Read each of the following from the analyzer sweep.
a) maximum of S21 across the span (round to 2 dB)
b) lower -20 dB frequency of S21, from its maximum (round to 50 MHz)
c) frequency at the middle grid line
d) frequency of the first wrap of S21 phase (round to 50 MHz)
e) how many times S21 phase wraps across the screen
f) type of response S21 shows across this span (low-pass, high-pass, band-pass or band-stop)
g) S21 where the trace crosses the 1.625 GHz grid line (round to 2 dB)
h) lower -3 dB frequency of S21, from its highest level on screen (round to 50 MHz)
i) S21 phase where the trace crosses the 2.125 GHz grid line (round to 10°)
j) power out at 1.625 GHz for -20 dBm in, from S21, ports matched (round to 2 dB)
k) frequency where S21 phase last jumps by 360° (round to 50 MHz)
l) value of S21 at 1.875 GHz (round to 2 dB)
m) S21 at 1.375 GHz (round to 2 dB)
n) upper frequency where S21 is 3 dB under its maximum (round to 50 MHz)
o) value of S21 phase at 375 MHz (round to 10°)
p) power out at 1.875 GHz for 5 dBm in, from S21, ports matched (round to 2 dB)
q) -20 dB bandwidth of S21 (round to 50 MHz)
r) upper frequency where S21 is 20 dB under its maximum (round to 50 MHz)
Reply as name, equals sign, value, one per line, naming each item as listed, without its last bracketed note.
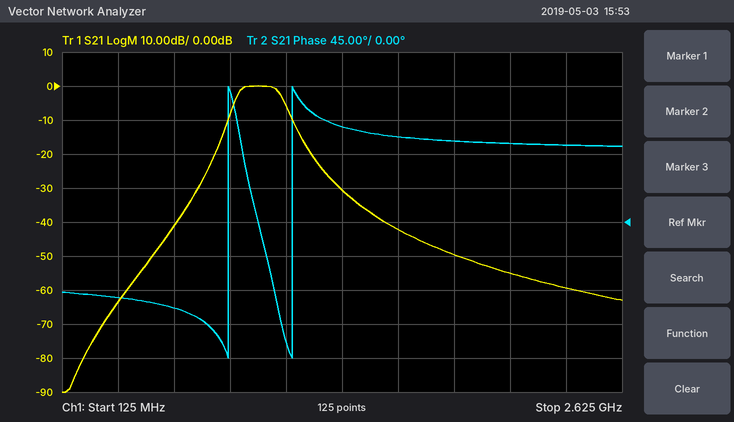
maximum of S21 across the span = 0 dB
lower -20 dB frequency of S21, from its maximum = 800 MHz
frequency at the middle grid line = 1.375 GHz
frequency of the first wrap of S21 phase = 850 MHz
how many times S21 phase wraps across the screen = 2
type of response S21 shows across this span = band-pass
S21 where the trace crosses the 1.625 GHz grid line = -42 dB
lower -3 dB frequency of S21, from its highest level on screen = 900 MHz
S21 phase where the trace crosses the 2.125 GHz grid line = 100°
power out at 1.625 GHz for -20 dBm in, from S21, ports matched = -62 dBm
frequency where S21 phase last jumps by 360° = 1.15 GHz
value of S21 at 1.875 GHz = -50 dB
S21 at 1.375 GHz = -30 dB
upper frequency where S21 is 3 dB under its maximum = 1.10 GHz
value of S21 phase at 375 MHz = -100°
power out at 1.875 GHz for 5 dBm in, from S21, ports matched = -44 dBm
-20 dB bandwidth of S21 = 450 MHz
upper frequency where S21 is 20 dB under its maximum = 1.25 GHz
